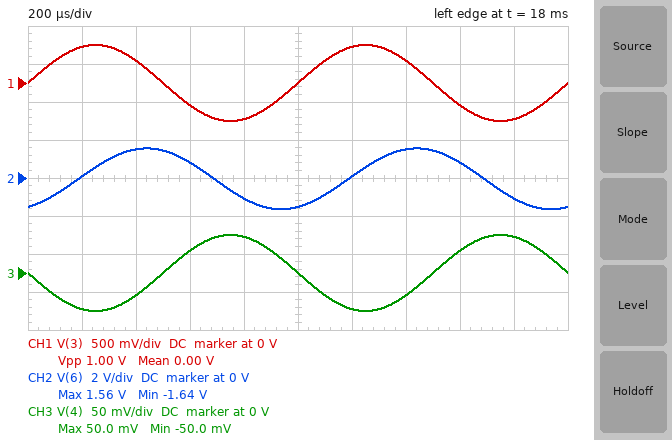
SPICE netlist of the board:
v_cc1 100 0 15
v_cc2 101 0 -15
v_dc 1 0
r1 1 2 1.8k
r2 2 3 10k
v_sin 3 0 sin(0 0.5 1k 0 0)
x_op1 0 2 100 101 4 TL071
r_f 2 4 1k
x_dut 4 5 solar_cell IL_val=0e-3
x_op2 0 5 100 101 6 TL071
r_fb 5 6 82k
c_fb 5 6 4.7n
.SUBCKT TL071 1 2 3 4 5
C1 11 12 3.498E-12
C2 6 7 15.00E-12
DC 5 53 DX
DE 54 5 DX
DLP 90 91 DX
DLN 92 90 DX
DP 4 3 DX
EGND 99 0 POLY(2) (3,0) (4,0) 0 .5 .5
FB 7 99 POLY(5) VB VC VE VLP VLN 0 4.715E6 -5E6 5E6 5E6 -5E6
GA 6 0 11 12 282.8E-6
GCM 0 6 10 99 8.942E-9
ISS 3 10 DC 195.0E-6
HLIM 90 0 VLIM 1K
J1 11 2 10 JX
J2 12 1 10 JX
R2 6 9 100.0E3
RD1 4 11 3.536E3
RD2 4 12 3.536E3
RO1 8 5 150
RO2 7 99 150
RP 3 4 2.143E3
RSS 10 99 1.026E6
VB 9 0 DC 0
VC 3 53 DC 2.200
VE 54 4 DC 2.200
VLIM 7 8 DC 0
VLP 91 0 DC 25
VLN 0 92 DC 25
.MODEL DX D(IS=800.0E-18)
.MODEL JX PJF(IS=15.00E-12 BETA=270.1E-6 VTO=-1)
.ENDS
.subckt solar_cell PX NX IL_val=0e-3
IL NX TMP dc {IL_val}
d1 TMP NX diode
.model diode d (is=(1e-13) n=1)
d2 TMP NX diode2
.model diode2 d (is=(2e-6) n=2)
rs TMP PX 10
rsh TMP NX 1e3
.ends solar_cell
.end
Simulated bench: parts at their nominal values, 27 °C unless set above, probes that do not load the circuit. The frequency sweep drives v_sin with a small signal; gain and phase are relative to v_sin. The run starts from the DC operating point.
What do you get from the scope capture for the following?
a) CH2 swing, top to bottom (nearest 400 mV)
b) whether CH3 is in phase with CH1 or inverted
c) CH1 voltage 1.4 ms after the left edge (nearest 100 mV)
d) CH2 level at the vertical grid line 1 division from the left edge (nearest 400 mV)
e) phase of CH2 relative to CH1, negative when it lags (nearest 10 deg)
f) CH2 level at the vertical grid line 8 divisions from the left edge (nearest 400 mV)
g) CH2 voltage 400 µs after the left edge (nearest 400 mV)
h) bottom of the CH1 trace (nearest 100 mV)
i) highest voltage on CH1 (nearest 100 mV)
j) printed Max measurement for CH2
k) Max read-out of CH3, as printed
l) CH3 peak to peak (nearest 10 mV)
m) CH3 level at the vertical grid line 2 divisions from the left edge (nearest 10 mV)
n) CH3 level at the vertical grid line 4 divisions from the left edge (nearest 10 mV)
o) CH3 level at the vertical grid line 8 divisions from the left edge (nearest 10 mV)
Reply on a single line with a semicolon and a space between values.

3.2 V; inverted; 300 mV; 0 V; -70 deg; 800 mV; 1.6 V; -500 mV; 500 mV; 1.56 V; 50.0 mV; 100 mV; -30 mV; 50 mV; 30 mV
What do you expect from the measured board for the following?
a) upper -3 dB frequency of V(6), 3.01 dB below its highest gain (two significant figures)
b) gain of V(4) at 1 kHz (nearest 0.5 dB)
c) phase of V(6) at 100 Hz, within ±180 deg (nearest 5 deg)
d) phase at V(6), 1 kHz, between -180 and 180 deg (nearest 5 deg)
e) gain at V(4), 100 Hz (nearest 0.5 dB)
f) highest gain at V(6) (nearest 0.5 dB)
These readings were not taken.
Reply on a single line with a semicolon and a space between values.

410 Hz; -20.0 dB; -15 deg; -70 deg; -20.0 dB; 18.5 dB
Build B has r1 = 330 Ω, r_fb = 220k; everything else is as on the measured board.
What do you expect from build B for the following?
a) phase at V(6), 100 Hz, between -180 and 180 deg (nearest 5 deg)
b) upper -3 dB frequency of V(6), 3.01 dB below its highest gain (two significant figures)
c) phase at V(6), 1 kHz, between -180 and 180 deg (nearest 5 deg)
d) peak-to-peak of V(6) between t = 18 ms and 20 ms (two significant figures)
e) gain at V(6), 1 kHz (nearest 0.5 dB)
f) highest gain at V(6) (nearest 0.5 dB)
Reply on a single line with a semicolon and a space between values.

-35 deg; 150 Hz; -80 deg; 3.4 V; 10.5 dB; 27.0 dB
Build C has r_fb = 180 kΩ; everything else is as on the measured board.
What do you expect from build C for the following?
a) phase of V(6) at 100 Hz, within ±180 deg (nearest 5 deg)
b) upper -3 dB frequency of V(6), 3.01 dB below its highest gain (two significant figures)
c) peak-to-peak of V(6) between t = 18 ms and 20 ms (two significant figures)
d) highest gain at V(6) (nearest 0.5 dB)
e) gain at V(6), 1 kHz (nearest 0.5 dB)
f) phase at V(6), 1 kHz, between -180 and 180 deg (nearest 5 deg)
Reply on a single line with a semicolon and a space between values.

-30 deg; 190 Hz; 3.4 V; 25.5 dB; 10.5 dB; -80 deg
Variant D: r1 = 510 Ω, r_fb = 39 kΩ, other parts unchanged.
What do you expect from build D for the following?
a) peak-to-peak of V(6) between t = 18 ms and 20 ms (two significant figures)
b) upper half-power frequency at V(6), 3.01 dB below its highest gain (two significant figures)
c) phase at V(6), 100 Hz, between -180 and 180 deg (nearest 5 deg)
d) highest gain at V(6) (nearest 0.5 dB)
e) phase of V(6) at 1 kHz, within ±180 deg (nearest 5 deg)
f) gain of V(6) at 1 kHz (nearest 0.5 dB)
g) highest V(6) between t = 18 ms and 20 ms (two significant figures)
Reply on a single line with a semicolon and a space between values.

2.6 V; 860 Hz; -5 deg; 12.0 dB; -50 deg; 8.5 dB; 1.3 V
